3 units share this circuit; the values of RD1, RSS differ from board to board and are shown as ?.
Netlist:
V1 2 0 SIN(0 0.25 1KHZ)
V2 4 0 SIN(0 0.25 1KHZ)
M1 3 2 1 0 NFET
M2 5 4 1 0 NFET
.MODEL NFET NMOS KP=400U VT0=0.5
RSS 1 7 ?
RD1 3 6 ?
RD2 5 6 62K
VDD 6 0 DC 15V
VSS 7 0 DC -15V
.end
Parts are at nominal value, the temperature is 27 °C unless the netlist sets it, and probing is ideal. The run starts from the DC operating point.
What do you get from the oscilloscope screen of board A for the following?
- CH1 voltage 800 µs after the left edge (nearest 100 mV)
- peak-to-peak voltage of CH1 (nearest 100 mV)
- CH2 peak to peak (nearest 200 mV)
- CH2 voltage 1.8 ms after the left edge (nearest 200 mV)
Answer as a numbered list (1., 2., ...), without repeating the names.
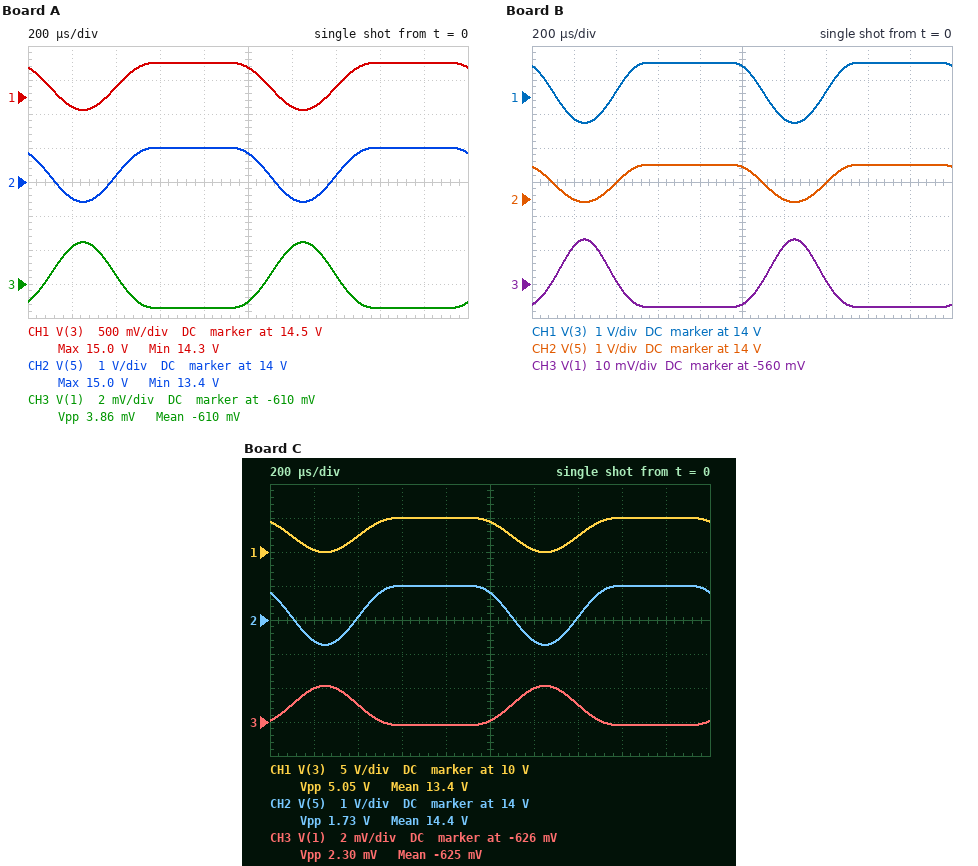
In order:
1. 15.0 V
2. 700 mV
3. 1.6 V
4. 15.0 V
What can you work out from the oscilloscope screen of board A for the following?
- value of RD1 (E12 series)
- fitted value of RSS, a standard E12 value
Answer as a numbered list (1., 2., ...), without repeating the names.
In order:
1. 27 kΩ
2. 39 kΩ
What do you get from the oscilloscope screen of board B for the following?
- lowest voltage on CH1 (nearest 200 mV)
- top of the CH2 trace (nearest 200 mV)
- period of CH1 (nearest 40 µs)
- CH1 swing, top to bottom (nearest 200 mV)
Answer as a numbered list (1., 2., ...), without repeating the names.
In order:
1. 13.2 V
2. 15.0 V
3. 1.00 ms
4. 1.8 V
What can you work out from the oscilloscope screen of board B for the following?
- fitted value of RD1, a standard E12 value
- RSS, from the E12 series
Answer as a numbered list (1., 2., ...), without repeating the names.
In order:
1. 100 kΩ
2. 220 kΩ
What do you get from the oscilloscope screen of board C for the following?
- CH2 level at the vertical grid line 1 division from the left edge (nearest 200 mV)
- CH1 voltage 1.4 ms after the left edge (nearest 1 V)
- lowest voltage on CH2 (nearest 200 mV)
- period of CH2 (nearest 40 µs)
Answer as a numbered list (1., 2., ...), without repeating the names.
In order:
1. 13.4 V
2. 12 V
3. 13.2 V
4. 1.00 ms
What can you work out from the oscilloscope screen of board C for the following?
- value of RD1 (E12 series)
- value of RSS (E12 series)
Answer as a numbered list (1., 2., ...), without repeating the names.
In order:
1. 180 kΩ
2. 22 kΩ
